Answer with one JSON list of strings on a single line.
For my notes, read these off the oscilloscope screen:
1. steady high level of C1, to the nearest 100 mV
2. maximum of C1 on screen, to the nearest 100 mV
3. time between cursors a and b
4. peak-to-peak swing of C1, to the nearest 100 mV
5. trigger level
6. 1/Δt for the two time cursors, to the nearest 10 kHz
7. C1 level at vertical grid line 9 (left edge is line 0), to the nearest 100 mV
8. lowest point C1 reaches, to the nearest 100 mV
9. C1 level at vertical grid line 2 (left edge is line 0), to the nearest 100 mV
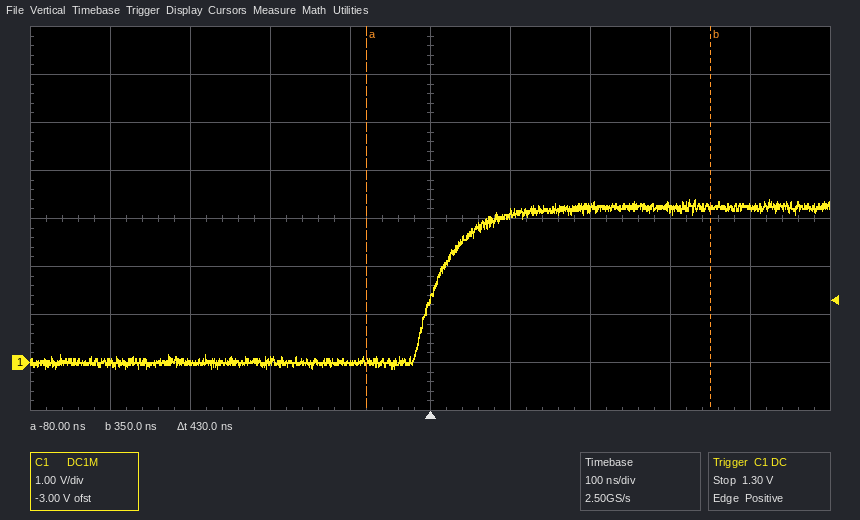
["3.2 V", "3.4 V", "430 ns", "3.5 V", "1.30 V", "2.33 MHz", "3.2 V", "-100 mV", "0.0 V"]
